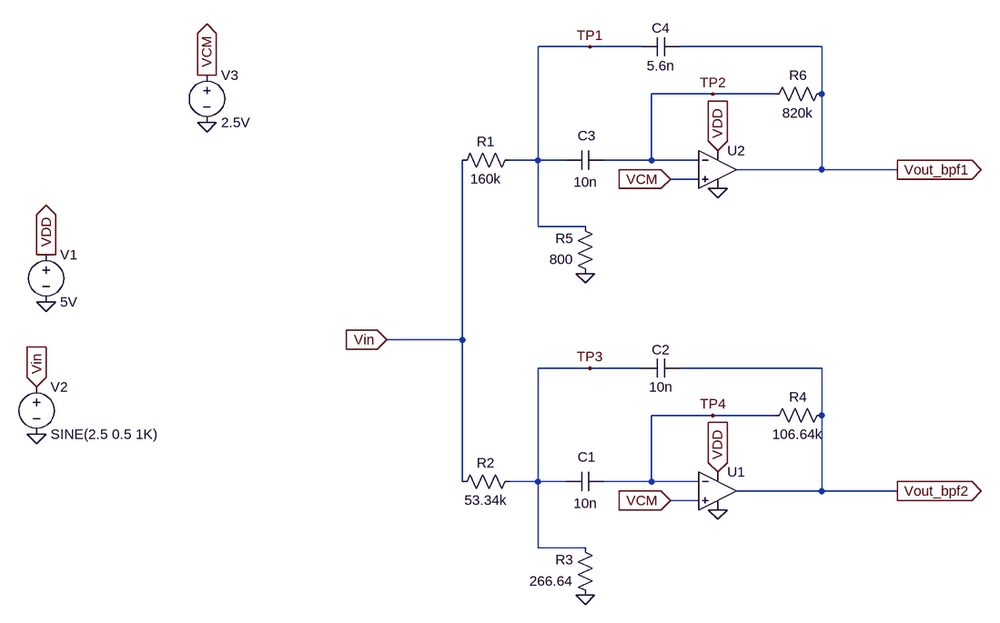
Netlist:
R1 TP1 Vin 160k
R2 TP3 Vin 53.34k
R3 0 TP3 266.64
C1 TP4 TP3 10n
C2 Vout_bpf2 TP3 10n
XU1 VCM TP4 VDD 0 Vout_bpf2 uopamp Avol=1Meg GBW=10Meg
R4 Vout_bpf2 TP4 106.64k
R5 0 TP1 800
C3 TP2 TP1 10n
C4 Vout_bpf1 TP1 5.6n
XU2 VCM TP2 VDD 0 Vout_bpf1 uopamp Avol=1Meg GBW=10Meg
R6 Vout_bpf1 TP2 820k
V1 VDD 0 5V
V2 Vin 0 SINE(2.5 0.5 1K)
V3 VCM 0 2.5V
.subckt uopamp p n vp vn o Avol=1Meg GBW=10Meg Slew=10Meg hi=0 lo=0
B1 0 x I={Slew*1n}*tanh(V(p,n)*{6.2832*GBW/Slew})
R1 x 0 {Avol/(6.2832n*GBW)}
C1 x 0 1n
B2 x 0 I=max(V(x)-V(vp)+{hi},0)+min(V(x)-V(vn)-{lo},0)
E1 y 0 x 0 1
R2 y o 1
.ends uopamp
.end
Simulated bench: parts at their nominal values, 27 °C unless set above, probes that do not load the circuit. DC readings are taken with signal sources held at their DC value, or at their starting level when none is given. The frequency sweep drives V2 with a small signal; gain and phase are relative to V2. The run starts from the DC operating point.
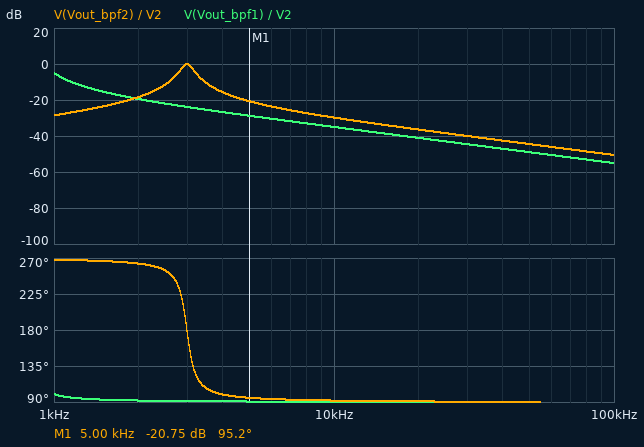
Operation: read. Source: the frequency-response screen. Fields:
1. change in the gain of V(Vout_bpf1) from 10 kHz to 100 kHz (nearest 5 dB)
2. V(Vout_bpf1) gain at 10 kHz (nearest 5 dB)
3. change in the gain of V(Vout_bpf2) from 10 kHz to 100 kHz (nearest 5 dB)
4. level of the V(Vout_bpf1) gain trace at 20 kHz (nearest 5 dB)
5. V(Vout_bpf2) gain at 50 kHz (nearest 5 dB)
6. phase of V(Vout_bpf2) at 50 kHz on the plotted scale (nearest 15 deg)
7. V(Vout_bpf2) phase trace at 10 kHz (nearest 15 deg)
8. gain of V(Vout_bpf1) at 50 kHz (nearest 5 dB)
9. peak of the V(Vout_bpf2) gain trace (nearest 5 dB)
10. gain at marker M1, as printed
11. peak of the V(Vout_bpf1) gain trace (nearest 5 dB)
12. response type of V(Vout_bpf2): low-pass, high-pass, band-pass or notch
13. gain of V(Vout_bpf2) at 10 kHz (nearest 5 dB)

-20 dB
-35 dB
-20 dB
-40 dB
-45 dB
90 deg
90 deg
-50 dB
0 dB
-20.75 dB
-5 dB
band-pass
-30 dB
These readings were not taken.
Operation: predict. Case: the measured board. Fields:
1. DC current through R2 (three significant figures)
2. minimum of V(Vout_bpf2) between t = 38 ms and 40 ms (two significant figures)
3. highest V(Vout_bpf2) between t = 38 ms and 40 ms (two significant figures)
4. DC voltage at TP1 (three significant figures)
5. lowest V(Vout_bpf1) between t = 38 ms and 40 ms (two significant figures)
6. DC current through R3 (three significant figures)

46.6 µA
2.5 V
2.5 V
12.4 mV
2.2 V
46.6 µA
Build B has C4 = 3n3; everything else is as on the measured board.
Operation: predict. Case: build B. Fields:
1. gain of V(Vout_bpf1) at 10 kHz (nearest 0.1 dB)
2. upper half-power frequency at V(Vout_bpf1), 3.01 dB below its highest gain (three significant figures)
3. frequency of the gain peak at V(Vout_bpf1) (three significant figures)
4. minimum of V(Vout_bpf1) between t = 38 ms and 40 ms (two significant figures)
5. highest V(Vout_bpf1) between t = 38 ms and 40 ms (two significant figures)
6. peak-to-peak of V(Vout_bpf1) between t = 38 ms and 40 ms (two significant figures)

-30.4 dB
1.12 kHz
1.08 kHz
1.7 V
3.3 V
1.6 V
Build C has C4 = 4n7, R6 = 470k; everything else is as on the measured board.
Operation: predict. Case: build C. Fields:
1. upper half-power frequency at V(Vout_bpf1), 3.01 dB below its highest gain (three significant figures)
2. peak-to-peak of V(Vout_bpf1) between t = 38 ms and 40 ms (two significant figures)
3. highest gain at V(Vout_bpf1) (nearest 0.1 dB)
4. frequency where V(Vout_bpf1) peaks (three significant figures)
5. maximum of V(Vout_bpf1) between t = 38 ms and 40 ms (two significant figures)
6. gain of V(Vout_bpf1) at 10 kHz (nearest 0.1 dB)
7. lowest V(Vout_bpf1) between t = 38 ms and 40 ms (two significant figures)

1.25 kHz
470 mV
6.0 dB
1.20 kHz
2.7 V
-33.4 dB
2.3 V
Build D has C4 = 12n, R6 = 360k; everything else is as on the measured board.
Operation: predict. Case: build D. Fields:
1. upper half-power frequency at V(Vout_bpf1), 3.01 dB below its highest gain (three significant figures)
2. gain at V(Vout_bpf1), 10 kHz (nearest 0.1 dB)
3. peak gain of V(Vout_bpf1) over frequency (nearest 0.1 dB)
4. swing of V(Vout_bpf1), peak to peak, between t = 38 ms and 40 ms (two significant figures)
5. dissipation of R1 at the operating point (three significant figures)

899 Hz
-41.6 dB
0.2 dB
300 mV
38.7 µW
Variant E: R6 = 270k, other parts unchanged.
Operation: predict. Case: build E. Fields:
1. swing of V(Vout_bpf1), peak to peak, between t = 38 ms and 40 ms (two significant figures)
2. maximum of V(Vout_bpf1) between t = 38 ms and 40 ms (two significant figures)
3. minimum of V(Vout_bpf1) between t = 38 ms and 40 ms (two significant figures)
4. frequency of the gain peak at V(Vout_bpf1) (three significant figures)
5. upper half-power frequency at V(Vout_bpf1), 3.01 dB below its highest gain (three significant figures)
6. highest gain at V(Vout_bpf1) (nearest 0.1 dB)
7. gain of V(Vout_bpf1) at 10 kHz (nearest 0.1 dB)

160 mV
2.6 V
2.4 V
1.45 kHz
1.53 kHz
0.7 dB
-34.9 dB
